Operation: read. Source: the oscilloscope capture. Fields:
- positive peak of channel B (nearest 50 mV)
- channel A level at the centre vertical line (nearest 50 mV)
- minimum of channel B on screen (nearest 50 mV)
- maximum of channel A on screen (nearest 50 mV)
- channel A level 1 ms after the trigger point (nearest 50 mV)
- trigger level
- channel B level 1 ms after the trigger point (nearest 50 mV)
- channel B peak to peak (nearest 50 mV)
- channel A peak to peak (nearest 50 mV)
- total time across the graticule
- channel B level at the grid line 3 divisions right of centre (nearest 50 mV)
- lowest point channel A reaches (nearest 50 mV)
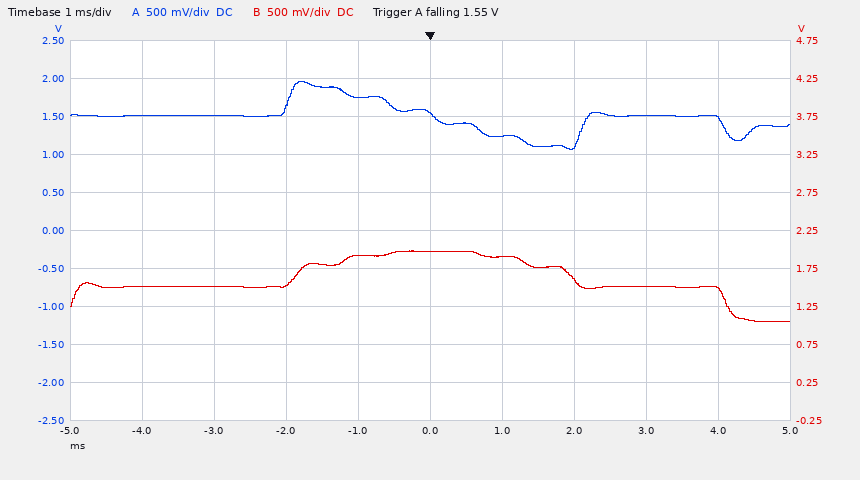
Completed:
2.00 V
1.55 V
1.05 V
1.95 V
1.25 V
1.55 V
1.90 V
950 mV
900 mV
10 ms
1.50 V
1.05 V
